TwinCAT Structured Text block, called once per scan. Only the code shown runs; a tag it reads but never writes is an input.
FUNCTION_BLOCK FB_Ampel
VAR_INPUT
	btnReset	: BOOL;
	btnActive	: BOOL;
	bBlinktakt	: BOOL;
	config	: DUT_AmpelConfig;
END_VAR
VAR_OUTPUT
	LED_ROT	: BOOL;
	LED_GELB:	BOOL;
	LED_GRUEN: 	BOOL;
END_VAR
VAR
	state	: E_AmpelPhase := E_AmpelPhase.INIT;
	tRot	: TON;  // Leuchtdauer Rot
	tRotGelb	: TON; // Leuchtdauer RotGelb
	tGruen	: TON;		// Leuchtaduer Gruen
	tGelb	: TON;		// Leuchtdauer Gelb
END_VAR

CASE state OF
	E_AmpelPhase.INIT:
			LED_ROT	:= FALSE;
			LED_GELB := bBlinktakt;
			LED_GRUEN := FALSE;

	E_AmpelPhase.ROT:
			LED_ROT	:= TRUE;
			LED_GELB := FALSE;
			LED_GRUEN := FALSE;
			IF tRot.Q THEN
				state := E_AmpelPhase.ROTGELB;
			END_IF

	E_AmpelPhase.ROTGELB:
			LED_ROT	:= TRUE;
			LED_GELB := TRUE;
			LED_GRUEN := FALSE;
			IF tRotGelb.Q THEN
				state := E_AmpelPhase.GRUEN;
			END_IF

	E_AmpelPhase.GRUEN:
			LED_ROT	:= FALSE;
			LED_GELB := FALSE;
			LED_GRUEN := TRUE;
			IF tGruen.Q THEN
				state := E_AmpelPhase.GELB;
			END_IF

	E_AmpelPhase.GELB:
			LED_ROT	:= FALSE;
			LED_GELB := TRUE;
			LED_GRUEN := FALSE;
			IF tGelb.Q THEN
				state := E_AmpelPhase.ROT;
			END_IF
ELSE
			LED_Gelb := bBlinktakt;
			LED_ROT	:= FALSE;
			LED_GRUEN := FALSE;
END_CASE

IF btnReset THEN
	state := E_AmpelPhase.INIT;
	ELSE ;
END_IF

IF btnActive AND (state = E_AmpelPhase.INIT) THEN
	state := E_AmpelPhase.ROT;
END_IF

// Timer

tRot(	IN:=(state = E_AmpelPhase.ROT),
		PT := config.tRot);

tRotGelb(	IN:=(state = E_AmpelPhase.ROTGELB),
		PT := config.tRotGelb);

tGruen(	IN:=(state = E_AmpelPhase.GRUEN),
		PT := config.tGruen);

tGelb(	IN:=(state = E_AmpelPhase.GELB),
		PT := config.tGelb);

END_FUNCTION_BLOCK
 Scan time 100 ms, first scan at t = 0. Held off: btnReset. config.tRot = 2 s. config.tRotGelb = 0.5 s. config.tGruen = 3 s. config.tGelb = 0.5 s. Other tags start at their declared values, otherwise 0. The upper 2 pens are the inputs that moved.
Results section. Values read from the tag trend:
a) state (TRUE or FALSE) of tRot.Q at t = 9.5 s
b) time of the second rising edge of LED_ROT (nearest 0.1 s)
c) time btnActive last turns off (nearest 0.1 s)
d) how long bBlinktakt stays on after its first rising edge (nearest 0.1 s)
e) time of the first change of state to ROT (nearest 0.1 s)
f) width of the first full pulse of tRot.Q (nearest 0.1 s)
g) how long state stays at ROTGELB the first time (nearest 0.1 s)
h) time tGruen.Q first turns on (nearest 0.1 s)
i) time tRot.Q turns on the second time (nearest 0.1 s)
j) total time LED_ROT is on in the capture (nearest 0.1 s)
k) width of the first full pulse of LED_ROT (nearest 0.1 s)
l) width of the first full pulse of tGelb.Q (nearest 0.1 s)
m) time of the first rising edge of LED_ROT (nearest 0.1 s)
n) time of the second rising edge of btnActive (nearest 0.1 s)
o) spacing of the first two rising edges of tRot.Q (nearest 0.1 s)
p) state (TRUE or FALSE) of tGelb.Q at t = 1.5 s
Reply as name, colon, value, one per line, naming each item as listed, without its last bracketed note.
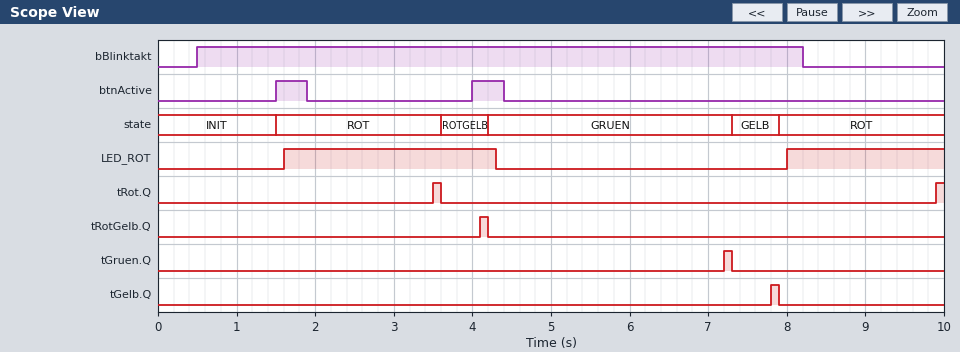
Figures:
state (TRUE or FALSE) of tRot.Q at t = 9.5 s: FALSE
time of the second rising edge of LED_ROT: 8.0 s
time btnActive last turns off: 4.4 s
how long bBlinktakt stays on after its first rising edge: 7.7 s
time of the first change of state to ROT: 1.5 s
width of the first full pulse of tRot.Q: 0.1 s
how long state stays at ROTGELB the first time: 0.6 s
time tGruen.Q first turns on: 7.2 s
time tRot.Q turns on the second time: 9.9 s
total time LED_ROT is on in the capture: 4.7 s
width of the first full pulse of LED_ROT: 2.7 s
width of the first full pulse of tGelb.Q: 0.1 s
time of the first rising edge of LED_ROT: 1.6 s
time of the second rising edge of btnActive: 4.0 s
spacing of the first two rising edges of tRot.Q: 6.4 s
state (TRUE or FALSE) of tGelb.Q at t = 1.5 s: FALSE
